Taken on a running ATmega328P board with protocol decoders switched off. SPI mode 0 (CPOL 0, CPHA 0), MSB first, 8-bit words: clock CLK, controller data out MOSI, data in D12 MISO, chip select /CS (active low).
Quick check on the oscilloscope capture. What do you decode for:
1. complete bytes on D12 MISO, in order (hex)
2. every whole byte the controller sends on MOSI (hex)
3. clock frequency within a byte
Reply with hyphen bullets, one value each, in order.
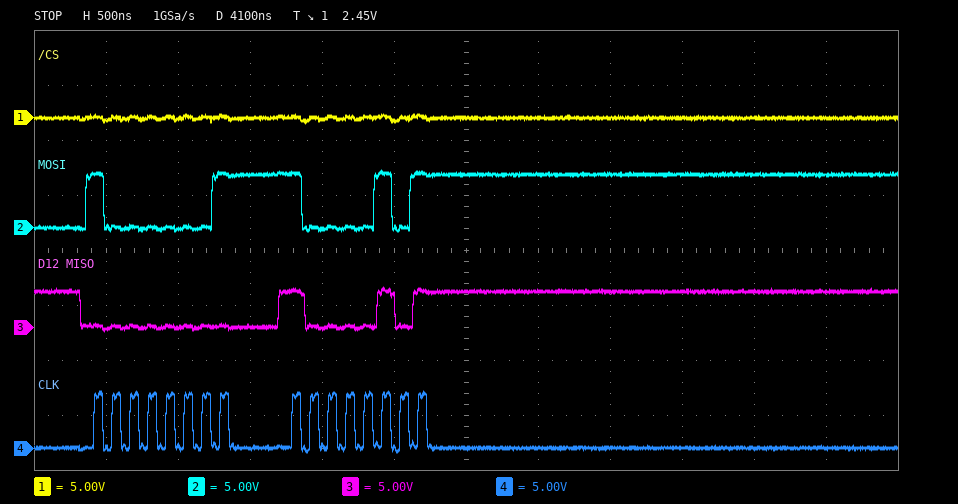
- 0x00 0x85
- 0x81 0x85
- 8 MHz
